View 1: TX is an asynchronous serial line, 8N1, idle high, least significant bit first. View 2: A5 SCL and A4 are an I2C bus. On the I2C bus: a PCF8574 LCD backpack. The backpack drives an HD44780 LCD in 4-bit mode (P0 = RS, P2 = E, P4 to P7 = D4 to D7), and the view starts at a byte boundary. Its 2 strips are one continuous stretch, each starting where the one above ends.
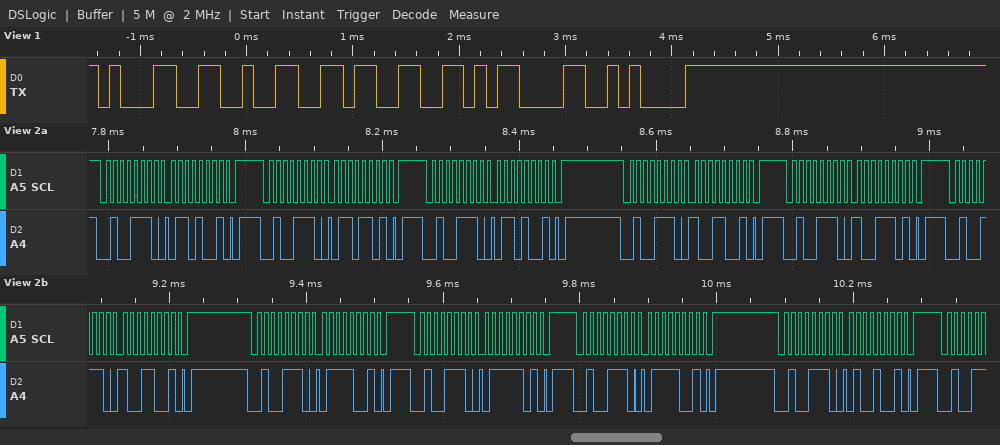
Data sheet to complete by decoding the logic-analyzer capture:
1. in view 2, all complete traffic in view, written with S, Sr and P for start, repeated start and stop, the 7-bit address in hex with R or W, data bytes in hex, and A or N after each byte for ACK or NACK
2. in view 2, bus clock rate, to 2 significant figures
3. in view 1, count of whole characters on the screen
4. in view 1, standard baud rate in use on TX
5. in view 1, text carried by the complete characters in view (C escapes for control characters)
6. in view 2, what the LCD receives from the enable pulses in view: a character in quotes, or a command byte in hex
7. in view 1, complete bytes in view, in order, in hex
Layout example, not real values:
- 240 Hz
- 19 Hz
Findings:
- S 27W A 69 A P S 27W A 6D A P S 27W A 69 A P S 27W A 99 A P S 27W A 9D A P S 27W A 99 A P S 27W A 79 A P S 27W A 7D A P S 27W A 79 A P S 27W A 49 A P
- 100 kHz
- 5
- 9600 baud
- "123\r\n"
- 'i'
- 31 32 33 0D 0A
